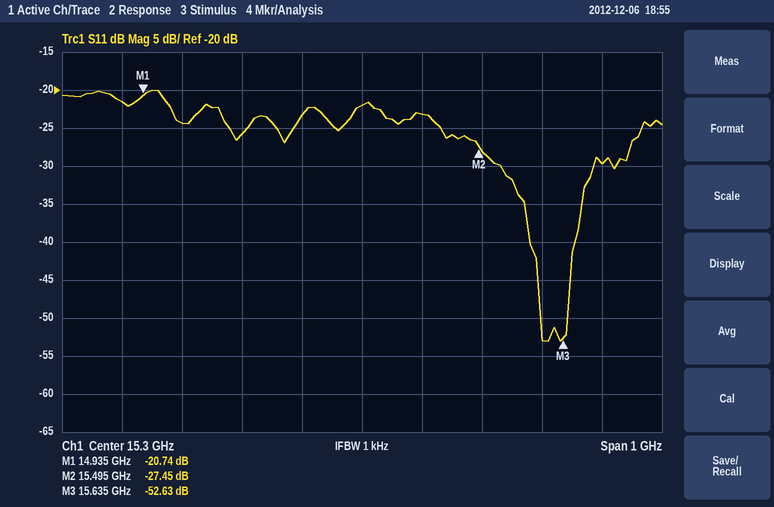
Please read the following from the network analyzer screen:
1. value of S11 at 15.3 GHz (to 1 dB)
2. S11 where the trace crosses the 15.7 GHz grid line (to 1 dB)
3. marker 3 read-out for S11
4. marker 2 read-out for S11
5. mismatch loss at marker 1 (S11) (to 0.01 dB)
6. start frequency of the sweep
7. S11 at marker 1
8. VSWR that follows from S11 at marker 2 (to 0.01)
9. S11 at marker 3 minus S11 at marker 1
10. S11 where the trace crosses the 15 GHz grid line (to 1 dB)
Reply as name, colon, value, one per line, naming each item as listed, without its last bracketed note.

value of S11 at 15.3 GHz: -22 dB
S11 where the trace crosses the 15.7 GHz grid line: -30 dB
marker 3 read-out for S11: -52.63 dB
marker 2 read-out for S11: -27.45 dB
mismatch loss at marker 1 (S11): 0.04 dB
start frequency of the sweep: 14.8 GHz
S11 at marker 1: -20.74 dB
VSWR that follows from S11 at marker 2: 1.09
S11 at marker 3 minus S11 at marker 1: -31.89 dB
S11 where the trace crosses the 15 GHz grid line: -24 dB
